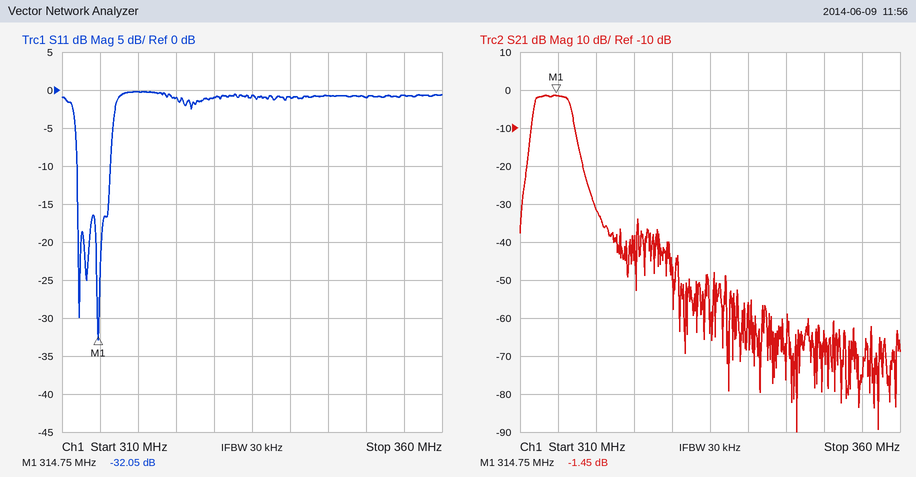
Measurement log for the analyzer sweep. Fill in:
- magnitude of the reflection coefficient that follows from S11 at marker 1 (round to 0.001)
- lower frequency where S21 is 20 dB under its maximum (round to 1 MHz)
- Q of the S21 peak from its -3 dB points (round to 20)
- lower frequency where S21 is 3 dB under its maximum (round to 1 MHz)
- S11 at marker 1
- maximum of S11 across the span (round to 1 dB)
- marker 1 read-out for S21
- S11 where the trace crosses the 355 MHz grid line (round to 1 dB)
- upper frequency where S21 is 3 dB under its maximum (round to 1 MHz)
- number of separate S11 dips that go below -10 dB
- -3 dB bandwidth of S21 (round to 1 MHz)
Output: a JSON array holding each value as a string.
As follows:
["0.025", "311 MHz", "60", "312 MHz", "-32.05 dB", "0 dB", "-1.45 dB", "-1 dB", "317 MHz", "3", "5 MHz"]
